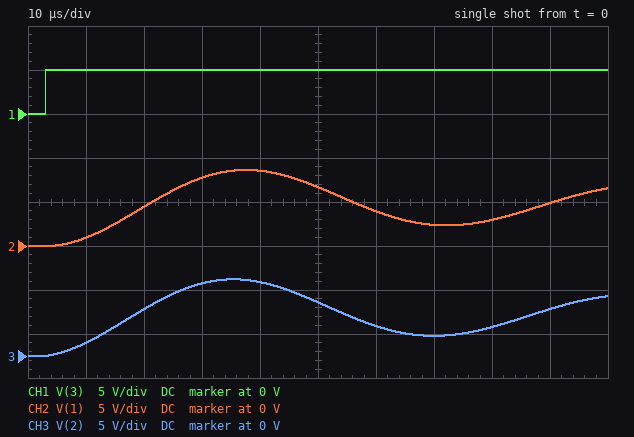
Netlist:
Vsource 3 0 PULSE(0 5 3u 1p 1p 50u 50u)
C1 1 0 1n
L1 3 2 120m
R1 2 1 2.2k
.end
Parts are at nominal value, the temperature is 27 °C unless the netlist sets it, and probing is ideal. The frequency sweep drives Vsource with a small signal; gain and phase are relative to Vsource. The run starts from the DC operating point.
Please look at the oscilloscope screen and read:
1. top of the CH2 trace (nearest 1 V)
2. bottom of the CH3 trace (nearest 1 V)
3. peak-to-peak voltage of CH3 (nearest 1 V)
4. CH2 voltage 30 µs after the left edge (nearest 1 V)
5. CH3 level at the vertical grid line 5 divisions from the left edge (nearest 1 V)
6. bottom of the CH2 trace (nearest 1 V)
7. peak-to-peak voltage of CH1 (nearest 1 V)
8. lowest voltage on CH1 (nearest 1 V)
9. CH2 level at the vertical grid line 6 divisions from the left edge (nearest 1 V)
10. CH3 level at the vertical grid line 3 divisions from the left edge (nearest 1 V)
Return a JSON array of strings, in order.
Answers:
["9 V", "0 V", "9 V", "8 V", "6 V", "0 V", "5 V", "0 V", "4 V", "8 V"]
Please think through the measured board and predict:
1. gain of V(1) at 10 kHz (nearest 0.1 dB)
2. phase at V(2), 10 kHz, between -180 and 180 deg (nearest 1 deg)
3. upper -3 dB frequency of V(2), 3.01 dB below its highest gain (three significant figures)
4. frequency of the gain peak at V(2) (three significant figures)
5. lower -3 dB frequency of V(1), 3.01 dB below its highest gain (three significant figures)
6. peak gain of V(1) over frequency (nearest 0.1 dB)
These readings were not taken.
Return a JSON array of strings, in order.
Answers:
["5.3 dB", "-7 deg", "15.8 kHz", "14.4 kHz", "12.8 kHz", "14.0 dB"]
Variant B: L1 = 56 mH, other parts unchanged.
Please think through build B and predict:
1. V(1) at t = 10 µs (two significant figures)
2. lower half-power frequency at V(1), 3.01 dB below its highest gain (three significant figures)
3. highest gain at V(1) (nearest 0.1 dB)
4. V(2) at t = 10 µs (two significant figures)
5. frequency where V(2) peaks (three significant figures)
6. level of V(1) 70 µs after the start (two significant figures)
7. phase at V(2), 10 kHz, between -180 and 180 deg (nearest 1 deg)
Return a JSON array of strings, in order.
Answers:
["1.9 V", "17.4 kHz", "10.7 dB", "2.9 V", "20.8 kHz", "6.0 V", "-2 deg"]
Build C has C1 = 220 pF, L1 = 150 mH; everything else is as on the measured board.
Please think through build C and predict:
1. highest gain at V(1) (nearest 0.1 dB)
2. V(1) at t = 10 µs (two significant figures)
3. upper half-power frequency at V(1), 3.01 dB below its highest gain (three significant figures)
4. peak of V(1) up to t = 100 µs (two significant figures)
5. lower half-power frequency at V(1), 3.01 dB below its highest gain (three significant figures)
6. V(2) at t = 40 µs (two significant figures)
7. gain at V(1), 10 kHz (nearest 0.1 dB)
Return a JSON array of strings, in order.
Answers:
["21.5 dB", "3.2 V", "28.8 kHz", "9.4 V", "26.5 kHz", "1.3 V", "1.2 dB"]
